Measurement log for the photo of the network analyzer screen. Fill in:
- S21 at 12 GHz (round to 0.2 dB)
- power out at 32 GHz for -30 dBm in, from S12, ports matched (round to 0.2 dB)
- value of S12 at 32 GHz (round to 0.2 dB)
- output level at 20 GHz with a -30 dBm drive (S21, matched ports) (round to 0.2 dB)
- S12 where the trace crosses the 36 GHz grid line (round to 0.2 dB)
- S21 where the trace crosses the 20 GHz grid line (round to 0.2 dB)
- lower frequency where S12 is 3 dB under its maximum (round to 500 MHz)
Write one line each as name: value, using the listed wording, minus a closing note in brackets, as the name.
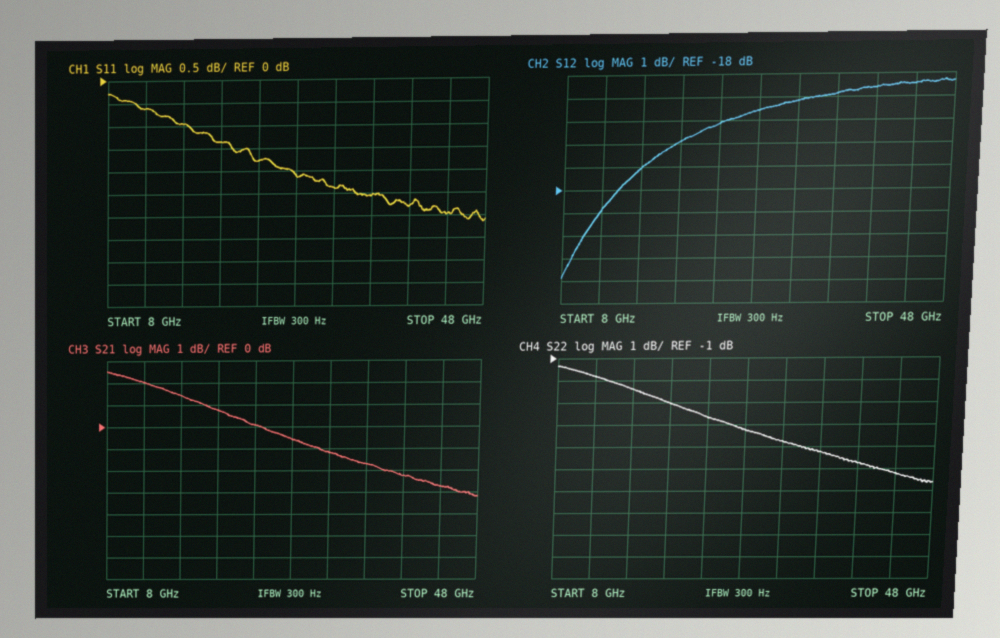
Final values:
S21 at 12 GHz: 2.0 dB
power out at 32 GHz for -30 dBm in, from S12, ports matched: -44.2 dBm
value of S12 at 32 GHz: -14.2 dB
output level at 20 GHz with a -30 dBm drive (S21, matched ports): -29.2 dBm
S12 where the trace crosses the 36 GHz grid line: -13.8 dB
S21 where the trace crosses the 20 GHz grid line: 0.8 dB
lower frequency where S12 is 3 dB under its maximum: 18.5 GHz
